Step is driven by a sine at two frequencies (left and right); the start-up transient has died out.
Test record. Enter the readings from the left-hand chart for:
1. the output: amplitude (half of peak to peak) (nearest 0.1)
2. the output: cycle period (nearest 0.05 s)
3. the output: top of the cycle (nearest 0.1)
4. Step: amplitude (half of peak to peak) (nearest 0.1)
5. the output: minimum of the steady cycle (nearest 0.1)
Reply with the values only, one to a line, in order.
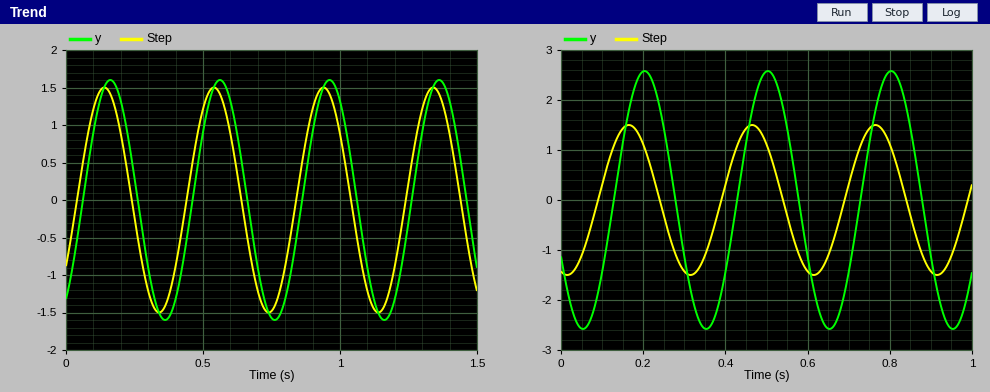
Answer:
1.6
0.40 s
1.6
1.5
-1.6
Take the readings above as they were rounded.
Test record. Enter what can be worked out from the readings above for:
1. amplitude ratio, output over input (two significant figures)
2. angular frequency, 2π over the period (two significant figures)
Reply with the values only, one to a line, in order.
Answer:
1.1
16 rad/s
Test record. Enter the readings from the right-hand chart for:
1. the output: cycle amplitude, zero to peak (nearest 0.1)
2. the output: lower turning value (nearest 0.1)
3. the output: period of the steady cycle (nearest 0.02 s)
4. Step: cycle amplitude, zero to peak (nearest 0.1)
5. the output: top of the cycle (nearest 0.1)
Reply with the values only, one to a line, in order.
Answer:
2.6
-2.6
0.30 s
1.5
2.6
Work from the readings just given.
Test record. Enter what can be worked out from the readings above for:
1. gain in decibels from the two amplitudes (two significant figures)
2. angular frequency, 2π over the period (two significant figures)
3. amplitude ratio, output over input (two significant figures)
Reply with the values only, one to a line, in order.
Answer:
4.8 dB
21 rad/s
1.7
